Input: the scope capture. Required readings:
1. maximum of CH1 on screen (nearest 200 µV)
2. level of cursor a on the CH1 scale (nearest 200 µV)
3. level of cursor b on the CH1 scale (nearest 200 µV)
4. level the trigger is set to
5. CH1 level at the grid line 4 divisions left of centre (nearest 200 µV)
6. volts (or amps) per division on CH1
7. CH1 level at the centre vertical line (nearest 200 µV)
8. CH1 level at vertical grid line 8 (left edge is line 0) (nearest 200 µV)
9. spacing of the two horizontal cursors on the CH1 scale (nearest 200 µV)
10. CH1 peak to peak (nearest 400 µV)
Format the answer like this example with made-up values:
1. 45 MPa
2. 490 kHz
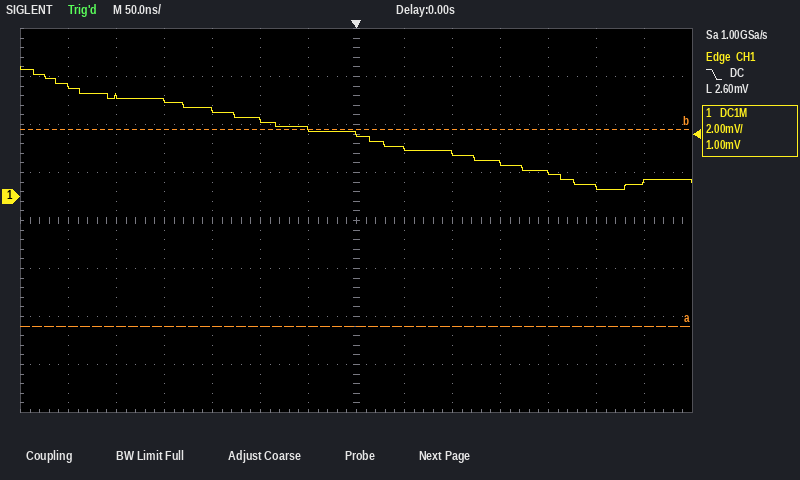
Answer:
1. 5.4 mV
2. -5.4 mV
3. 2.8 mV
4. 2.60 mV
5. 4.0 mV
6. 2 mV
7. 2.6 mV
8. 2.0 mV
9. 8.2 mV
10. 5.2 mV
